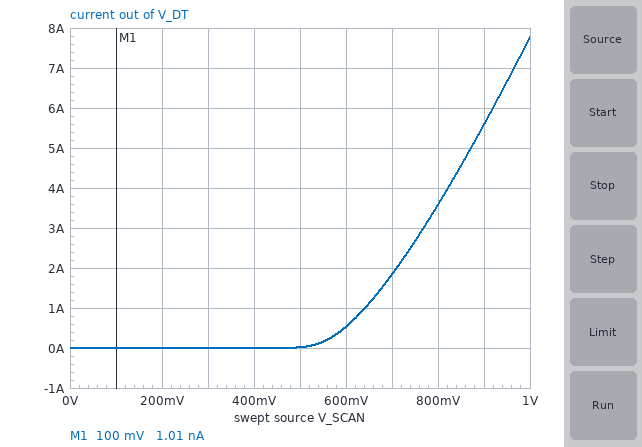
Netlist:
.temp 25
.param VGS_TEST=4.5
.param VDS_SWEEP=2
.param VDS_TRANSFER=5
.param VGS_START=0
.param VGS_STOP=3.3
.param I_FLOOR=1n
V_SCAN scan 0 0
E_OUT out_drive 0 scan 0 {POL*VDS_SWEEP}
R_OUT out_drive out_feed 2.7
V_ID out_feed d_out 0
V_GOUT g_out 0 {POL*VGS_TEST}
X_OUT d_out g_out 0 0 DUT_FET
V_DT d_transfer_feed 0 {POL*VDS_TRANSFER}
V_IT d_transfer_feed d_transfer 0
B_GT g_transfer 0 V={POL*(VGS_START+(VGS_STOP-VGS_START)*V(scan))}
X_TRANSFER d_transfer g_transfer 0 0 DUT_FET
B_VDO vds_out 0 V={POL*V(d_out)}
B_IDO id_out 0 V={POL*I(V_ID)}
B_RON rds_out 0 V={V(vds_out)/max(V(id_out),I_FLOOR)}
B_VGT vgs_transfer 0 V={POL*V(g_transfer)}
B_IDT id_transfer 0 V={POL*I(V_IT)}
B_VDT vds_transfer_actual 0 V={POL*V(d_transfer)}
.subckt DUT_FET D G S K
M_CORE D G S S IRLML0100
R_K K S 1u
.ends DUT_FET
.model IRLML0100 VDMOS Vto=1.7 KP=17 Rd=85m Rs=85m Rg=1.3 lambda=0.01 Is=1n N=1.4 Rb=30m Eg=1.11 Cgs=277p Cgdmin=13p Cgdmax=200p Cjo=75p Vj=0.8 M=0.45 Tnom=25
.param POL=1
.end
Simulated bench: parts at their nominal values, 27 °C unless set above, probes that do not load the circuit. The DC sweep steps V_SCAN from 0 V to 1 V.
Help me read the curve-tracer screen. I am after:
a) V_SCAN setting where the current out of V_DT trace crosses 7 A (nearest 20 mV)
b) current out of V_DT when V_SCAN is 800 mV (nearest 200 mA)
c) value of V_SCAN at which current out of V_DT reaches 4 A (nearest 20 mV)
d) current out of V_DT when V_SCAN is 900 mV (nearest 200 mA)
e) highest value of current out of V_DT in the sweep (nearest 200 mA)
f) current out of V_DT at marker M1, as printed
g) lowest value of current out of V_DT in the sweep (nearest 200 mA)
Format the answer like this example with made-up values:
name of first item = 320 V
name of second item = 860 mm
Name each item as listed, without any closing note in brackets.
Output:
V_SCAN setting where the current out of V_DT trace crosses 7 A = 960 mV
current out of V_DT when V_SCAN is 800 mV = 3.6 A
value of V_SCAN at which current out of V_DT reaches 4 A = 820 mV
current out of V_DT when V_SCAN is 900 mV = 5.6 A
highest value of current out of V_DT in the sweep = 7.8 A
current out of V_DT at marker M1, as printed = 1.01 nA
lowest value of current out of V_DT in the sweep = 0 A
